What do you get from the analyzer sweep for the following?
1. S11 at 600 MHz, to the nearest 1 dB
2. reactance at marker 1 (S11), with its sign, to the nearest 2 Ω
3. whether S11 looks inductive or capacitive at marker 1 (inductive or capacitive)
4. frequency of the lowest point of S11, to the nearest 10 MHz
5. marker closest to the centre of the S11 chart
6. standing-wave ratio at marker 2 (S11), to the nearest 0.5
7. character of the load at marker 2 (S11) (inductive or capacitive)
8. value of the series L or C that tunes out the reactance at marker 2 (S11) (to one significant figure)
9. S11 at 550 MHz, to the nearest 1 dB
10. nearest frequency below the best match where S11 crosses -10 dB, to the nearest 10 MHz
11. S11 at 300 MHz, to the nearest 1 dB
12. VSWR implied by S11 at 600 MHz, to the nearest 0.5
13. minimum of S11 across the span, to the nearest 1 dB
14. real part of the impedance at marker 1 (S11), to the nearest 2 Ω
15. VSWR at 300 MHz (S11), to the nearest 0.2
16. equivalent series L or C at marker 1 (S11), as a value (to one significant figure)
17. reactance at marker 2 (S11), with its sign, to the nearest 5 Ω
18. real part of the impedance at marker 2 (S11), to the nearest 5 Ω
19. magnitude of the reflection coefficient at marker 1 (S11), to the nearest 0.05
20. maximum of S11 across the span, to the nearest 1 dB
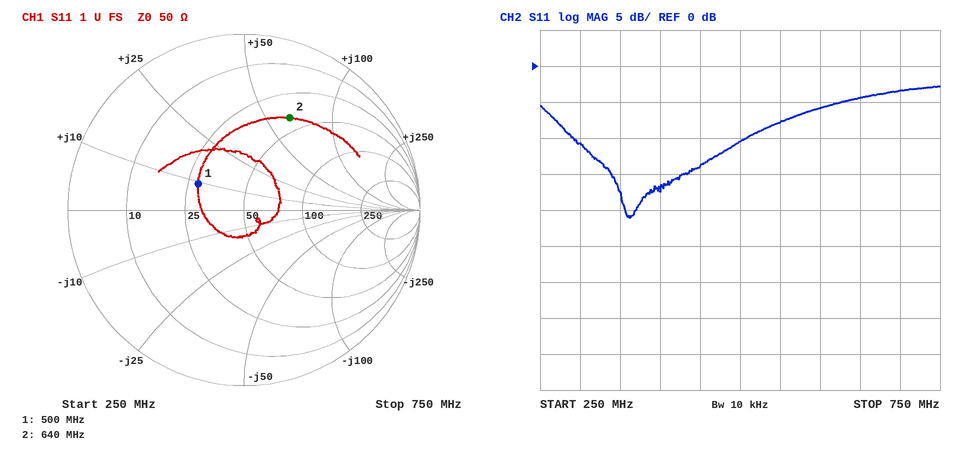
-6 dB
+10 Ω
inductive
360 MHz
marker 1
4.0
inductive
4 pF
-8 dB
290 MHz
-11 dB
3.0
-21 dB
28 Ω
1.8
3 nH
+65 Ω
40 Ω
0.30
-3 dB
